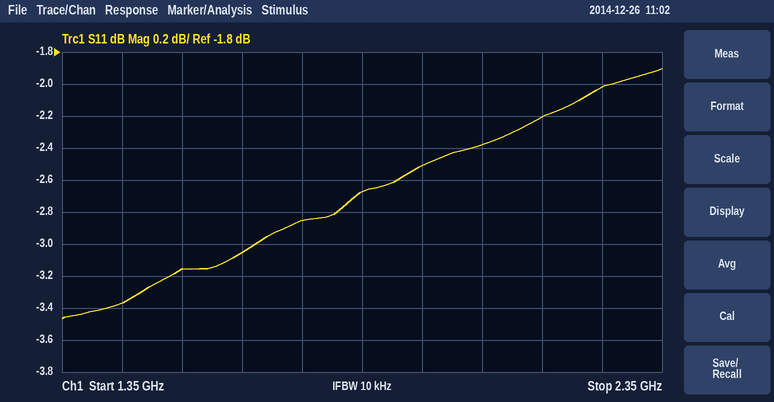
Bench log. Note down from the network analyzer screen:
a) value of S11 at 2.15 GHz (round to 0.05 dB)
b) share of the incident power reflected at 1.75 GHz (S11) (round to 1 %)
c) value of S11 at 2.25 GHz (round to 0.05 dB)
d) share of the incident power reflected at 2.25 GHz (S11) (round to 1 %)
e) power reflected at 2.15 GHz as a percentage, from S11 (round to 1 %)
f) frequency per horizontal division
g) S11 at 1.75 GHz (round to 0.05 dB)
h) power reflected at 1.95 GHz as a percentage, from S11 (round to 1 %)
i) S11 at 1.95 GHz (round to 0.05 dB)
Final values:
-2.20 dB
52 %
-2.00 dB
63 %
60 %
100 MHz
-2.85 dB
56 %
-2.50 dB
